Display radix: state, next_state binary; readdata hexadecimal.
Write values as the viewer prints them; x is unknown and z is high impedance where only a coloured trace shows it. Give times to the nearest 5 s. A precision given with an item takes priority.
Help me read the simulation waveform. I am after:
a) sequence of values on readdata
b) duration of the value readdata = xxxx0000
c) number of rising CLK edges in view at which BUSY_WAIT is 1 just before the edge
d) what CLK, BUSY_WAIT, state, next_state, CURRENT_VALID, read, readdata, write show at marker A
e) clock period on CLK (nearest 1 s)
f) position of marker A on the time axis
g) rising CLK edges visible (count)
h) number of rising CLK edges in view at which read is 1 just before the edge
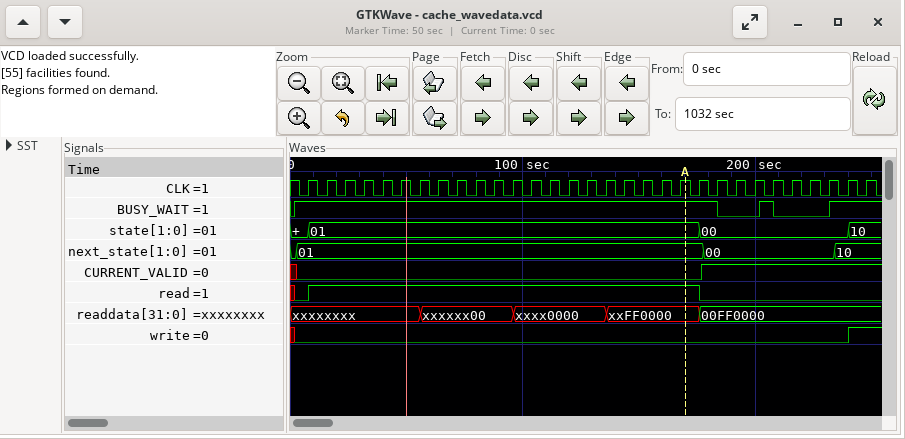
xxxxxxxx, xxxxxx00, xxxx0000, xxFF0000, 00FF0000
40 s
26
CLK=1, BUSY_WAIT=1, state=01, next_state=01, CURRENT_VALID=0, read=1, readdata=xxFF0000, write=0
8 s
170 s
31
21
